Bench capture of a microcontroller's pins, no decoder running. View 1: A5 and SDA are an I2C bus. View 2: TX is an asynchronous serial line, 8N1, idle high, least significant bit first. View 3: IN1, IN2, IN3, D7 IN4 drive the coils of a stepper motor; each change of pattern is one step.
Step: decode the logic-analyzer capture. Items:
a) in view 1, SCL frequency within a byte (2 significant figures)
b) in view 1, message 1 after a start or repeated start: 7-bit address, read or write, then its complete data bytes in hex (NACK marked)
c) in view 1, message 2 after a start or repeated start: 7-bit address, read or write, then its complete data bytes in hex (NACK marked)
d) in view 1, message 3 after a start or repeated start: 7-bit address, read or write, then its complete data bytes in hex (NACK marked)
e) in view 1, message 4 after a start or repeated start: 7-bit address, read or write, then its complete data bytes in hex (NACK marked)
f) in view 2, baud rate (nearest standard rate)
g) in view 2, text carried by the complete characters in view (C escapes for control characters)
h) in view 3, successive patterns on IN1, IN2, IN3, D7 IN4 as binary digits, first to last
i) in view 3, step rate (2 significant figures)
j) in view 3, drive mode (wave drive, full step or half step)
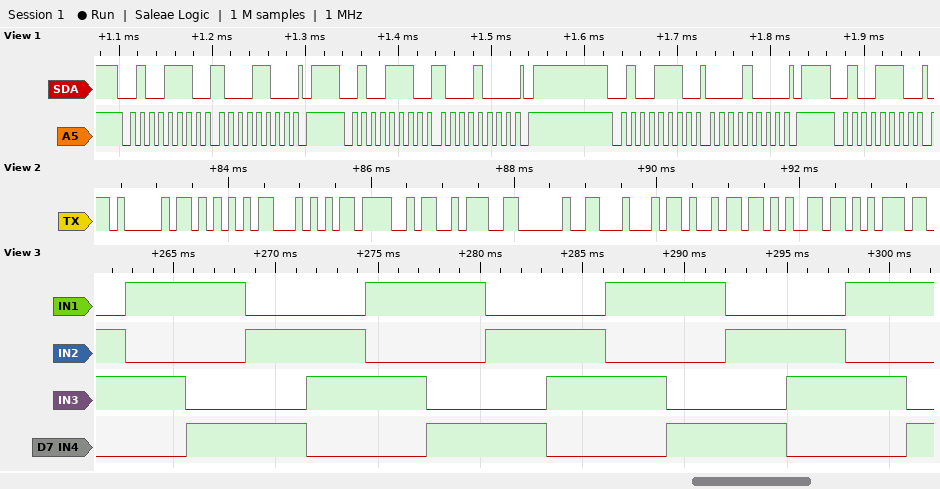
100 kHz
0x27 write: 8C
0x27 write: 88
0x27 write: 08
0x27 write
9600 baud
"AUTO: Dieu"
0110 1010 1001 0101 0110 1010 1001 0101 0110 1010 1001 0101 0110 1010 1001
340 steps/s
full step
